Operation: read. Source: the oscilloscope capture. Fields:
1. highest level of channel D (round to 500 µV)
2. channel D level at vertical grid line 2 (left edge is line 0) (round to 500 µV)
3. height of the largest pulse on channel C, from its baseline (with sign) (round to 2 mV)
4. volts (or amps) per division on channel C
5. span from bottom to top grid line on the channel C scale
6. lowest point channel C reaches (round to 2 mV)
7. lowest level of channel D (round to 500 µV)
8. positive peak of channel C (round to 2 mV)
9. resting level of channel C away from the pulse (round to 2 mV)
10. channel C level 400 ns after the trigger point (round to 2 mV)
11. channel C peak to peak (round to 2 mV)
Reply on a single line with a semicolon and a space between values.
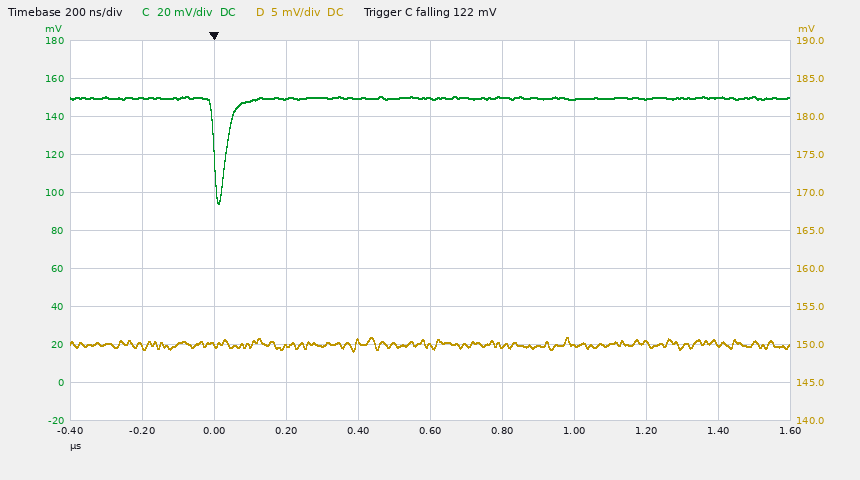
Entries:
151.0 mV; 150.0 mV; -56 mV; 20 mV; 200 mV; 94 mV; 149.0 mV; 150 mV; 150 mV; 150 mV; 56 mV
